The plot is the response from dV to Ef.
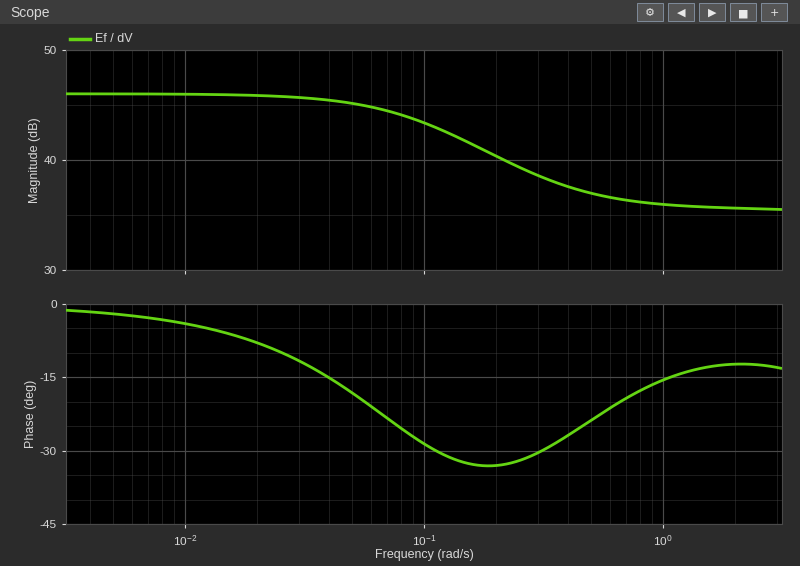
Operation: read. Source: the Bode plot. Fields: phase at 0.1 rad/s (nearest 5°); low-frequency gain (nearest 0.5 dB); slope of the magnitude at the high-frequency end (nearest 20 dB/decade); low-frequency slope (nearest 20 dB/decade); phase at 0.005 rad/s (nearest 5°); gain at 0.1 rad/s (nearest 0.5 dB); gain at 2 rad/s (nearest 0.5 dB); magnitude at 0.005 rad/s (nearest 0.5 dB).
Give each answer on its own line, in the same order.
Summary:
-30°
46.0 dB
0 dB/decade
0 dB/decade
0°
43.5 dB
35.5 dB
46.0 dB
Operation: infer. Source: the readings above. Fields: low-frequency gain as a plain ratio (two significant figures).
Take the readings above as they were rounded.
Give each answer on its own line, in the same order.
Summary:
200
